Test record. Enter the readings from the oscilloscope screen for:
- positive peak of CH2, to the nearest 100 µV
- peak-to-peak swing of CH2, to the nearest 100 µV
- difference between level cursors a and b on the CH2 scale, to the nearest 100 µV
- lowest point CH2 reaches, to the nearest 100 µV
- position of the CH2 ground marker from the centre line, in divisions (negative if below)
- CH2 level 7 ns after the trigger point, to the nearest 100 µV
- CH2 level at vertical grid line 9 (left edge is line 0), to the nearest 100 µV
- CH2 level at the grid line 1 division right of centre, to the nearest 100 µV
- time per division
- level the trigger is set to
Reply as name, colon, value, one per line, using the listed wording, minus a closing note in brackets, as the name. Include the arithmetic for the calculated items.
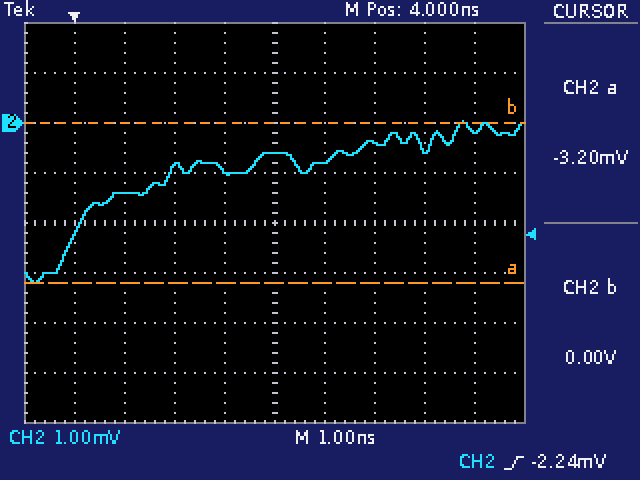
positive peak of CH2, to the nearest 100 µV: 0.0 mV
peak-to-peak swing of CH2, to the nearest 100 µV: 0.0 mV − (-3.2 mV) = 3.2 mV
difference between level cursors a and b on the CH2 scale, to the nearest 100 µV: 3.2 mV
lowest point CH2 reaches, to the nearest 100 µV: -3.2 mV
position of the CH2 ground marker from the centre line, in divisions: +2.0 div
CH2 level 7 ns after the trigger point, to the nearest 100 µV: -500 µV
CH2 level at vertical grid line 9 (left edge is line 0), to the nearest 100 µV: -200 µV
CH2 level at the grid line 1 division right of centre, to the nearest 100 µV: -800 µV
time per division: 1 ns
level the trigger is set to: -2.24 mV
